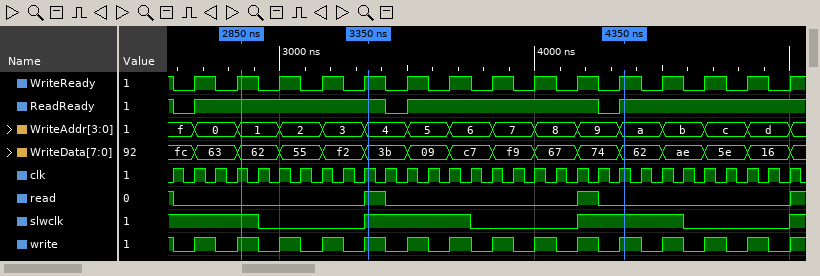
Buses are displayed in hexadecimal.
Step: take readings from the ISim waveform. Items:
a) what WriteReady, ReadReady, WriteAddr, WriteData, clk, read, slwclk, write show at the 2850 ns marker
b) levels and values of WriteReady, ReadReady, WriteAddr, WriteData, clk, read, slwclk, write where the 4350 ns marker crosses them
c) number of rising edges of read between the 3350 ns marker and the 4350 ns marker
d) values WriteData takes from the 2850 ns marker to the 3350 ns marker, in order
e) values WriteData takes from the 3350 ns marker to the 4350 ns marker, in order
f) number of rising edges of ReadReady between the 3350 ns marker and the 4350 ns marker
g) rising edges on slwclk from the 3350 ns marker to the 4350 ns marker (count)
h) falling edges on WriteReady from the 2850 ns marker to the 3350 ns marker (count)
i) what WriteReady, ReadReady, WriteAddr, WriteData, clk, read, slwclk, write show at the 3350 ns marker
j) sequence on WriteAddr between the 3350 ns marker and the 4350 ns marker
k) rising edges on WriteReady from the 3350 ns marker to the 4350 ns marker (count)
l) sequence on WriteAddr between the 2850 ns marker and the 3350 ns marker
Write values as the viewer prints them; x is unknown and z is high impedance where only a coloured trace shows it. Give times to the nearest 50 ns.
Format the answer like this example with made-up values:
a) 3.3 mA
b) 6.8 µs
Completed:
a) WriteReady=1, ReadReady=1, WriteAddr=1, WriteData=62, clk=1, read=0, slwclk=1, write=1
b) WriteReady=1, ReadReady=1, WriteAddr=a, WriteData=62, clk=1, read=0, slwclk=1, write=1
c) 1
d) 62, 55, f2, 3b
e) 3b, 09, c7, f9, 67, 74, 62
f) 2
g) 1
h) 3
i) WriteReady=1, ReadReady=1, WriteAddr=4, WriteData=3b, clk=1, read=1, slwclk=1, write=1
j) 4, 5, 6, 7, 8, 9, a
k) 6
l) 1, 2, 3, 4
